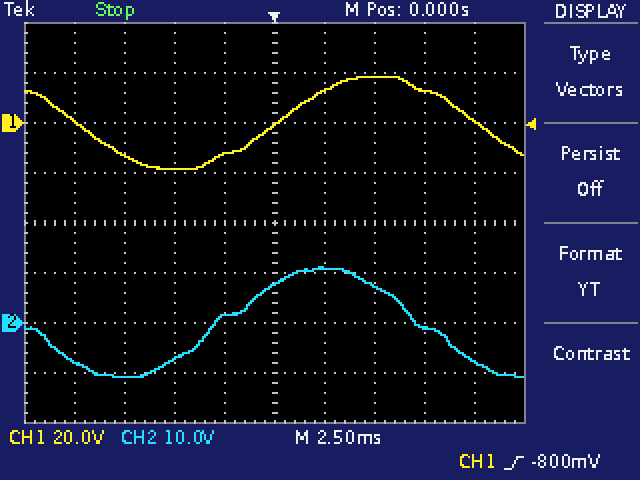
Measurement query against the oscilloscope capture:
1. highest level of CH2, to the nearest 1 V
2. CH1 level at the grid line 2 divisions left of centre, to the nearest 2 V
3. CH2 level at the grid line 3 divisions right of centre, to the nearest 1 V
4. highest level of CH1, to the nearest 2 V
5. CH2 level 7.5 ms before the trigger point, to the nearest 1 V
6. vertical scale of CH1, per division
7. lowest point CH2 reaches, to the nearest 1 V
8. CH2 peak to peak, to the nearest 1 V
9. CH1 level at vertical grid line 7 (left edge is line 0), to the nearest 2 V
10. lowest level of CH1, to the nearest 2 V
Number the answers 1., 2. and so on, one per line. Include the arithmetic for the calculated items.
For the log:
1. 11 V
2. -18 V
3. -1 V
4. 18 V
5. -11 V
6. 20 V
7. -11 V
8. 11 V − (-11 V) = 22 V
9. 18 V
10. -18 V
